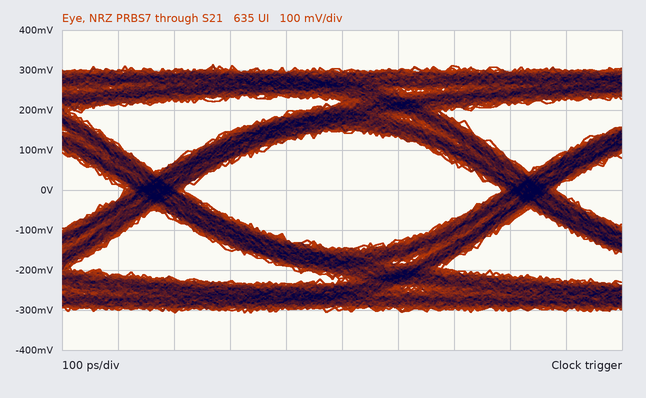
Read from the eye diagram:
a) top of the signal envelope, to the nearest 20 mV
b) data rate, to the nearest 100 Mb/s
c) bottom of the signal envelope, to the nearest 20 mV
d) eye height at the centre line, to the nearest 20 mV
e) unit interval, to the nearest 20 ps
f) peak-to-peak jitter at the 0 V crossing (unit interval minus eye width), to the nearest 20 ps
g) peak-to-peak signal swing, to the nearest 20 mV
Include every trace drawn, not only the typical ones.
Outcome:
320 mV
1.5 Gb/s
-300 mV
300 mV
660 ps
100 ps
620 mV
